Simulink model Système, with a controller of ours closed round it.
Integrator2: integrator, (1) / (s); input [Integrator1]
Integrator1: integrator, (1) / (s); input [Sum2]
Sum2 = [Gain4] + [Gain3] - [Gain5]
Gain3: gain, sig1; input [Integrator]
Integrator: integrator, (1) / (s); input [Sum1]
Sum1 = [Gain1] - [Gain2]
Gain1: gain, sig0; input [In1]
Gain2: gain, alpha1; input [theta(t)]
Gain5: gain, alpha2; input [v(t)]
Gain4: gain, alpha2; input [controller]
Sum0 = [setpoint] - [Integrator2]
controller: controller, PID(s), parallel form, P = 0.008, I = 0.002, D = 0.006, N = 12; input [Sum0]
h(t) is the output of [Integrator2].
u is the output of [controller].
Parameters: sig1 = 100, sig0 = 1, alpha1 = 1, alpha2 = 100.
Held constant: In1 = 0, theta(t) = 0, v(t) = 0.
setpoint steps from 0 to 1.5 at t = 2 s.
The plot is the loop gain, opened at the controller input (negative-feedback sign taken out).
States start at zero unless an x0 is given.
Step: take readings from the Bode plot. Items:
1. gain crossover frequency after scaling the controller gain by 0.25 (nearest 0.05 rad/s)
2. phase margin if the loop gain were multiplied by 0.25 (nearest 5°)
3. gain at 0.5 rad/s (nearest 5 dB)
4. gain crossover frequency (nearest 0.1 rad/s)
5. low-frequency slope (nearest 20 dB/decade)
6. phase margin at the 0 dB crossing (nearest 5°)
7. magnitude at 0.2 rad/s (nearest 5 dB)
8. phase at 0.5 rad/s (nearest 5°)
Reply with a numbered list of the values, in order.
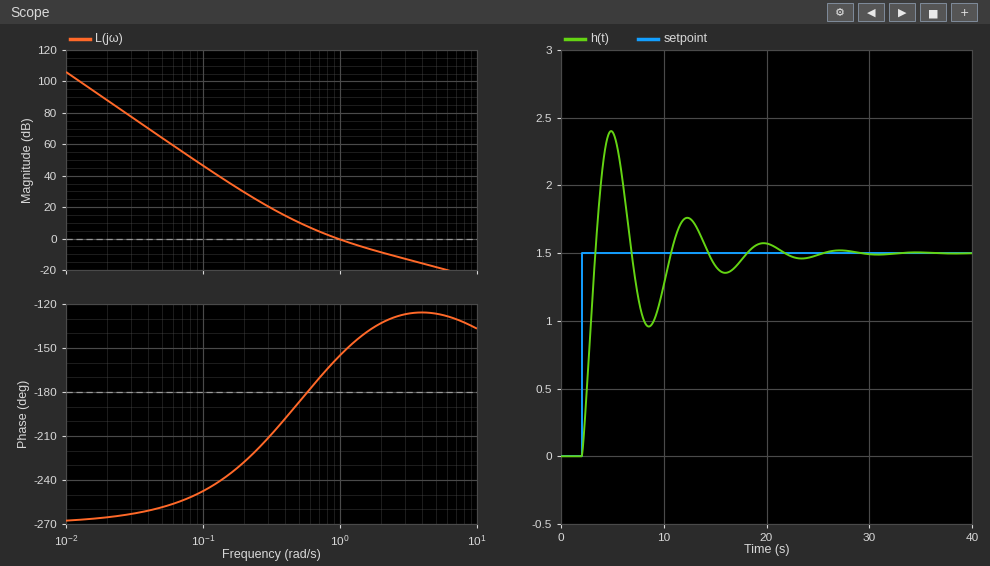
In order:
1. 0.45 rad/s
2. -10°
3. 10 dB
4. 1.0 rad/s
5. -60 dB/decade
6. 25°
7. 30 dB
8. -185°
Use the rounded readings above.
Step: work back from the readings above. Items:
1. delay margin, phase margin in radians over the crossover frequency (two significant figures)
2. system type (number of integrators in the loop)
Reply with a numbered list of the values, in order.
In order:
1. 0.44 s
2. 3
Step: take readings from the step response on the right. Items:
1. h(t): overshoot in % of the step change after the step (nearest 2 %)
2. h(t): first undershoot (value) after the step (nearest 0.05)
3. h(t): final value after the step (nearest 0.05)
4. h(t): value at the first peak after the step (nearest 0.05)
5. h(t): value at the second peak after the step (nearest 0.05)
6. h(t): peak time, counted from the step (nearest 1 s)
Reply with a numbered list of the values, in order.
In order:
1. 60 %
2. 0.95
3. 1.50
4. 2.40
5. 1.75
6. 3 s
